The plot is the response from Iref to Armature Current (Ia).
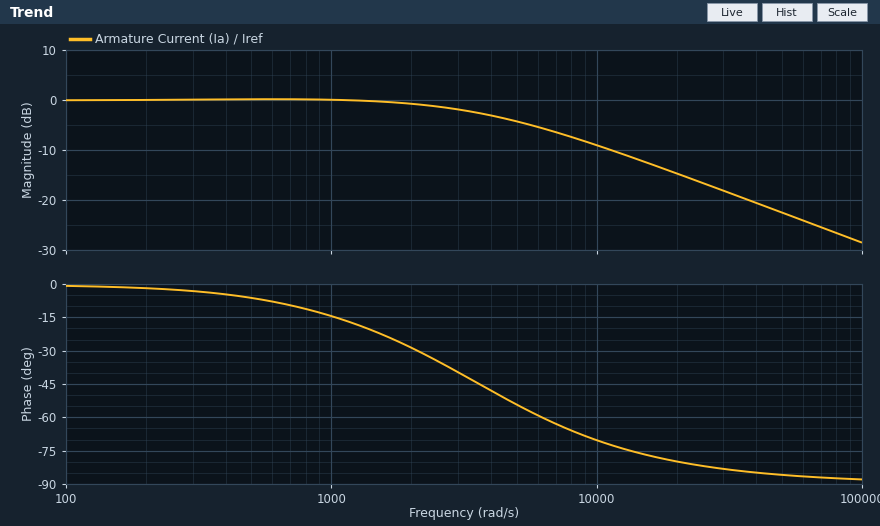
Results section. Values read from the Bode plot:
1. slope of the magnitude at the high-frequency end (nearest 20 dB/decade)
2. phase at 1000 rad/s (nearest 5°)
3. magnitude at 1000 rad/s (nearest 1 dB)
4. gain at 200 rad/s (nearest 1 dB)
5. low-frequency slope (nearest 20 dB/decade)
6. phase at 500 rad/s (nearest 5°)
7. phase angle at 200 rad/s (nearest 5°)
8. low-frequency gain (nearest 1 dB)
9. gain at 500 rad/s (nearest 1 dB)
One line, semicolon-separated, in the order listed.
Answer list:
-20 dB/decade; -15°; 0 dB; 0 dB; 0 dB/decade; -5°; 0°; 0 dB; 0 dB
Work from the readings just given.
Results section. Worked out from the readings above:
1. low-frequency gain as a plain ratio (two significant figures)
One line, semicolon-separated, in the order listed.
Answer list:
1.0
